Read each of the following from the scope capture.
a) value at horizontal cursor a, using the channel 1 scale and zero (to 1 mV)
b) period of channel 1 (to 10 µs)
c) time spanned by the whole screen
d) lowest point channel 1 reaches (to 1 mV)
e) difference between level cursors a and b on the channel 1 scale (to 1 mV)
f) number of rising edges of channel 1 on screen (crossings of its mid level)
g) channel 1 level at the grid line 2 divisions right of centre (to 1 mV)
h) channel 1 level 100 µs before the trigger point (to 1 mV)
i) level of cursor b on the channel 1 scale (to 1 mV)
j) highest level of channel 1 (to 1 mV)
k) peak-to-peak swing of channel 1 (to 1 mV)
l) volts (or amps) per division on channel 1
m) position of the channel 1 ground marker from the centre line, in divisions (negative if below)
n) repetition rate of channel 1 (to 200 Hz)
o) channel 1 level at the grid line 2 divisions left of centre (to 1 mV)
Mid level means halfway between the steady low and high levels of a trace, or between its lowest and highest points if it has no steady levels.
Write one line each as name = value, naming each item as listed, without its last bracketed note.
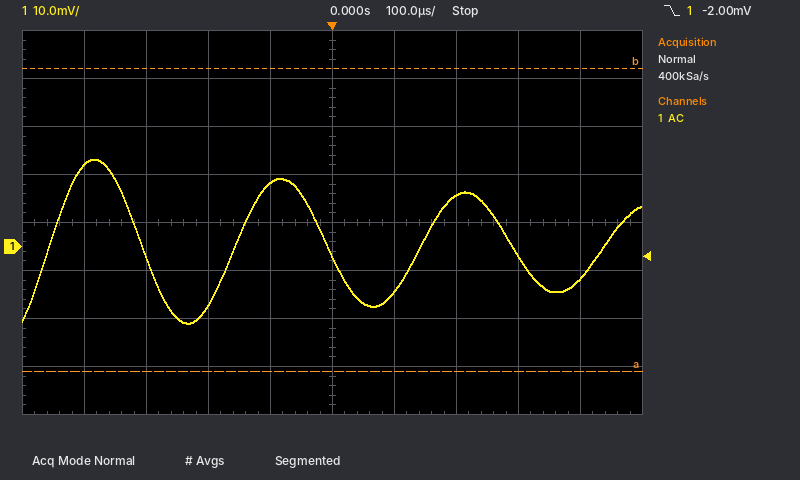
value at horizontal cursor a, using the channel 1 scale and zero = -26 mV
period of channel 1 = 300 µs
time spanned by the whole screen = 1 ms
lowest point channel 1 reaches = -16 mV
difference between level cursors a and b on the channel 1 scale = 63 mV
number of rising edges of channel 1 on screen = 4
channel 1 level at the grid line 2 divisions right of centre = 11 mV
channel 1 level 100 µs before the trigger point = 13 mV
level of cursor b on the channel 1 scale = 37 mV
highest level of channel 1 = 18 mV
peak-to-peak swing of channel 1 = 34 mV
volts (or amps) per division on channel 1 = 10 mV
position of the channel 1 ground marker from the centre line, in divisions = -0.5 div
repetition rate of channel 1 = 3.4 kHz
channel 1 level at the grid line 2 divisions left of centre = -12 mV
